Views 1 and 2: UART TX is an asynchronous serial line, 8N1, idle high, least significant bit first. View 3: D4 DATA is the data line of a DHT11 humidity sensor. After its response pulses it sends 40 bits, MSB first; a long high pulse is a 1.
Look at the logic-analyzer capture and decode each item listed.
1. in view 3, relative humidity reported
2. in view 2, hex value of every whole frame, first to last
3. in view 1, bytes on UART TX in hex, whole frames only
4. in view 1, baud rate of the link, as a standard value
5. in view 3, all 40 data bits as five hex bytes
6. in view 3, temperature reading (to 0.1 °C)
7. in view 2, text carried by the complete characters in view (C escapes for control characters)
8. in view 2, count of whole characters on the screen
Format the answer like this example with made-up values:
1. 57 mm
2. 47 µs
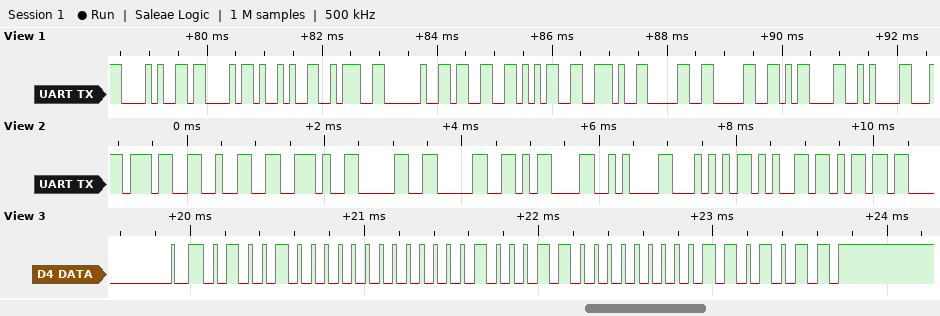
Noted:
1. 72 %
2. 0x37 0x32 0x2E 0x30 0x30 0x0D 0x0A 0x54 0x65 0x6D
3. 28 43 29 3A 20 33 35 2E 30 30 0D 0A
4. 9600 baud
5. 48 00 23 00 6B
6. 35.0 °C
7. "72.00\r\nTem"
8. 10
